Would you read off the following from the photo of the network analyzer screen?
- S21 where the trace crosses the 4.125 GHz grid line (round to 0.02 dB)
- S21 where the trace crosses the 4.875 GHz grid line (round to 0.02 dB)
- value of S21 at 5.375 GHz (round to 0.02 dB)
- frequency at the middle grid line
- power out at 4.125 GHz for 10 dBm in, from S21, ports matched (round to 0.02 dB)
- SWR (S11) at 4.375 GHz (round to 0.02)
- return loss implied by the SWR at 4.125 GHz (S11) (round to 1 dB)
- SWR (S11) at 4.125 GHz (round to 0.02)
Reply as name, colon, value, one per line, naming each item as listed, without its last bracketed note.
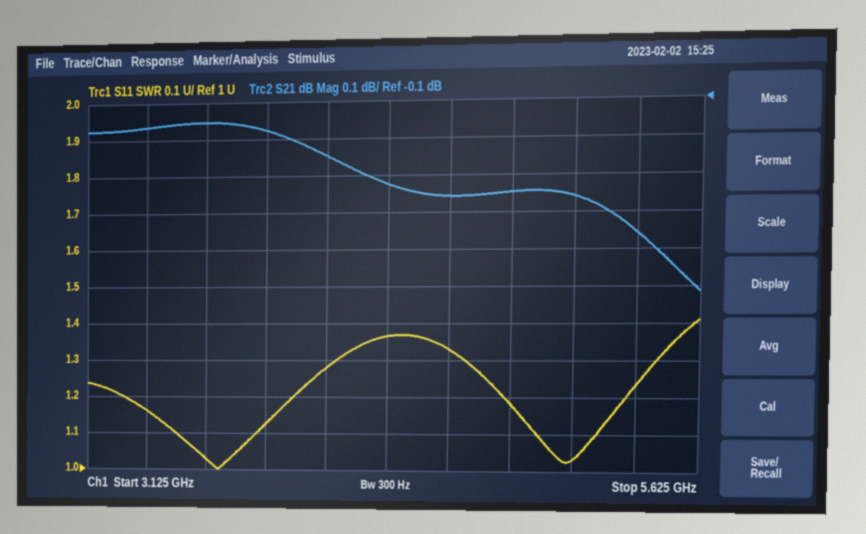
S21 where the trace crosses the 4.125 GHz grid line: -0.24 dB
S21 where the trace crosses the 4.875 GHz grid line: -0.34 dB
value of S21 at 5.375 GHz: -0.46 dB
frequency at the middle grid line: 4.375 GHz
power out at 4.125 GHz for 10 dBm in, from S21, ports matched: 9.76 dBm
SWR (S11) at 4.375 GHz: 1.36
return loss implied by the SWR at 4.125 GHz (S11): 18 dB
SWR (S11) at 4.125 GHz: 1.28
